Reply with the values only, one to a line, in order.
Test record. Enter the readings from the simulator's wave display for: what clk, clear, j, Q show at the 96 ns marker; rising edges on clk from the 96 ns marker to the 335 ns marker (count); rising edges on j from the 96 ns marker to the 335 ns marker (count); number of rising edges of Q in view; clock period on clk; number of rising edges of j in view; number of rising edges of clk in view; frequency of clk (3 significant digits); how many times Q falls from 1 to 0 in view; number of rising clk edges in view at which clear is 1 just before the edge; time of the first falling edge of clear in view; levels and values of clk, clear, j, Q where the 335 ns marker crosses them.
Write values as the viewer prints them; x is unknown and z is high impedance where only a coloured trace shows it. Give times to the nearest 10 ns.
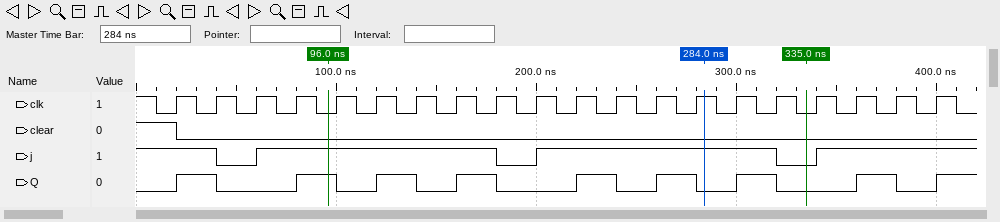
clk=0, clear=0, j=1, Q=1
12
1
9
20 ns
3
20
50.0 MHz
8
1
20 ns
clk=0, clear=0, j=0, Q=0
